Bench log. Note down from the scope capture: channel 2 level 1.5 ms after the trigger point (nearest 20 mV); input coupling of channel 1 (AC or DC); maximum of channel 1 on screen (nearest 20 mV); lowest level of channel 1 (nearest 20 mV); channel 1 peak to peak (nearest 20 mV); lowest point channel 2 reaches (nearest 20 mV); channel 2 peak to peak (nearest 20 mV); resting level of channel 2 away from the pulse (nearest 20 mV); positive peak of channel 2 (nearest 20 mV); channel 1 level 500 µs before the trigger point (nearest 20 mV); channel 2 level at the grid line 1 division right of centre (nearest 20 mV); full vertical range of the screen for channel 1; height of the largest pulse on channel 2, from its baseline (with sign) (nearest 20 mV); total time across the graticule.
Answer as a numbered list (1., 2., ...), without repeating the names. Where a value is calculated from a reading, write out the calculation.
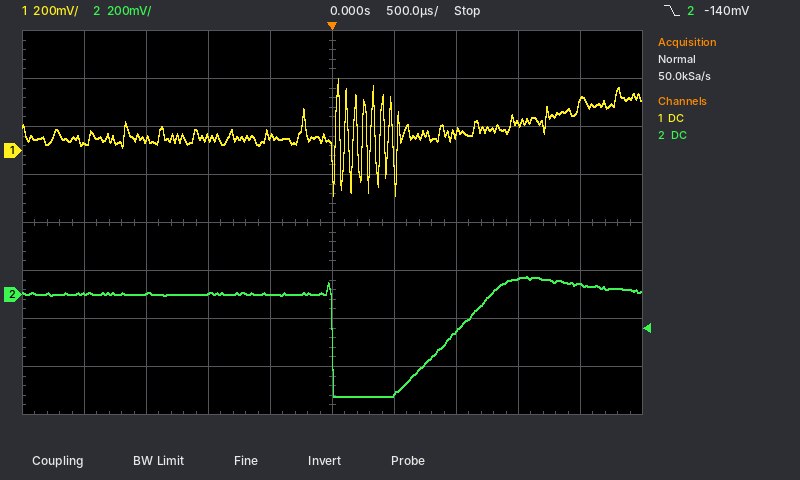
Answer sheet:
1. 60 mV
2. DC
3. 300 mV
4. -180 mV
5. 300 mV − (-180 mV) = 480 mV
6. -420 mV
7. 80 mV − (-420 mV) = 500 mV
8. 0 mV
9. 80 mV
10. 60 mV
11. -420 mV
12. 1.6 V
13. -420 mV − (0 mV) = -420 mV
14. 5 ms
